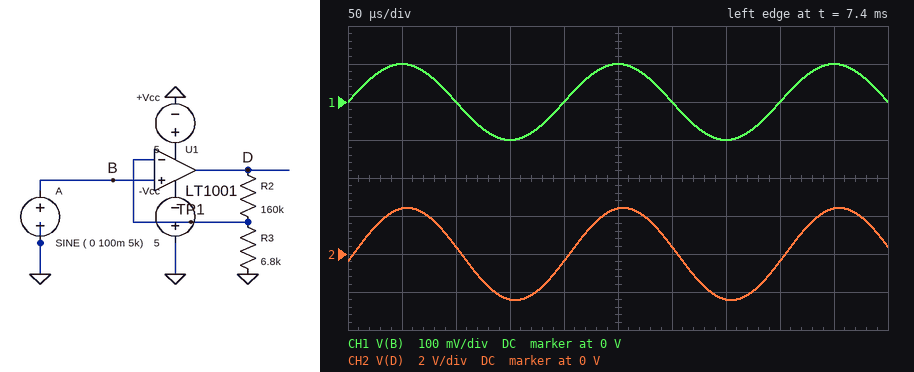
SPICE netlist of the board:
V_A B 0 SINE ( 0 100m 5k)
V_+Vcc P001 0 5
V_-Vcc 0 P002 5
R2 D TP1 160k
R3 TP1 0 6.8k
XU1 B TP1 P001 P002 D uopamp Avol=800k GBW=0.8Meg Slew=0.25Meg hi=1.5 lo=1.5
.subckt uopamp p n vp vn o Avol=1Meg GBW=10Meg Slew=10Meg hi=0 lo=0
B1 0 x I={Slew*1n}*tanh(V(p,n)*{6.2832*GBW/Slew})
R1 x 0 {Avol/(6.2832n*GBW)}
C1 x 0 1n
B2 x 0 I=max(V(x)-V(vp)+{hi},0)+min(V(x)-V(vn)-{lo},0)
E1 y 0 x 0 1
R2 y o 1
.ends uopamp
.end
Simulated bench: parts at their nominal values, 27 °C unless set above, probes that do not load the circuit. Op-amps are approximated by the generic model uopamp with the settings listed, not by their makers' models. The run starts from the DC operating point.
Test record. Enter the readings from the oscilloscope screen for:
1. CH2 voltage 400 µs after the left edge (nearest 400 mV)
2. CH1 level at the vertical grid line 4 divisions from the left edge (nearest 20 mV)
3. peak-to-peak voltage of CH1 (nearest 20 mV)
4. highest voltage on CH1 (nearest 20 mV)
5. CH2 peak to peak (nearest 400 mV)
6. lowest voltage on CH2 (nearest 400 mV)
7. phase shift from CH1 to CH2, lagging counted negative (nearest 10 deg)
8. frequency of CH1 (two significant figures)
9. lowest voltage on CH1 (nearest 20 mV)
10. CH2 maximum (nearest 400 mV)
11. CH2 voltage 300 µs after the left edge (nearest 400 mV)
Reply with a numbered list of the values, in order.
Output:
1. -400 mV
2. 0 V
3. 200 mV
4. 100 mV
5. 4.8 V
6. -2.4 V
7. -10 deg
8. 5.0 kHz
9. -100 mV
10. 2.4 V
11. 400 mV
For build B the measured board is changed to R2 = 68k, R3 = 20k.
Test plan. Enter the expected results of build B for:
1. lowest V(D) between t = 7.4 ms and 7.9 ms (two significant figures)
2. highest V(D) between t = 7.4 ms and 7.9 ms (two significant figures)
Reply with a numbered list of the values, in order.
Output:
1. -440 mV
2. 440 mV
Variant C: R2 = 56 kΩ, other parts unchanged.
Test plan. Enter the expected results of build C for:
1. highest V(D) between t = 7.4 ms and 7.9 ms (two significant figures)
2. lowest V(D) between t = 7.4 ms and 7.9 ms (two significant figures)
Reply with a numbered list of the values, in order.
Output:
1. 920 mV
2. -920 mV
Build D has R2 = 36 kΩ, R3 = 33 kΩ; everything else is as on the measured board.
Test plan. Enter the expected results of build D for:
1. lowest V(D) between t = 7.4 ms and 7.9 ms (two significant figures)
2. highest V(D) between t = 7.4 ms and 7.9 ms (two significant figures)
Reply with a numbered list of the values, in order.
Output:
1. -210 mV
2. 210 mV
